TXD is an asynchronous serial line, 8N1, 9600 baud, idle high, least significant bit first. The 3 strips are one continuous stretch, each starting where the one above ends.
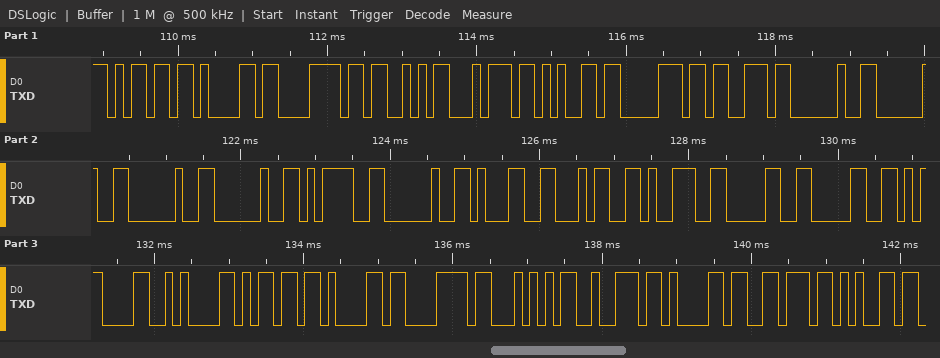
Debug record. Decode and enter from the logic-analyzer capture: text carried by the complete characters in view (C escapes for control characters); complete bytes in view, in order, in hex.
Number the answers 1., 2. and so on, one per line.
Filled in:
1. "maxSteps    = 14900\r\nmaxTrave"
2. 6D 61 78 53 74 65 70 73 20 20 20 20 3D 20 31 34 39 30 30 0D 0A 6D 61 78 54 72 61 76 65
